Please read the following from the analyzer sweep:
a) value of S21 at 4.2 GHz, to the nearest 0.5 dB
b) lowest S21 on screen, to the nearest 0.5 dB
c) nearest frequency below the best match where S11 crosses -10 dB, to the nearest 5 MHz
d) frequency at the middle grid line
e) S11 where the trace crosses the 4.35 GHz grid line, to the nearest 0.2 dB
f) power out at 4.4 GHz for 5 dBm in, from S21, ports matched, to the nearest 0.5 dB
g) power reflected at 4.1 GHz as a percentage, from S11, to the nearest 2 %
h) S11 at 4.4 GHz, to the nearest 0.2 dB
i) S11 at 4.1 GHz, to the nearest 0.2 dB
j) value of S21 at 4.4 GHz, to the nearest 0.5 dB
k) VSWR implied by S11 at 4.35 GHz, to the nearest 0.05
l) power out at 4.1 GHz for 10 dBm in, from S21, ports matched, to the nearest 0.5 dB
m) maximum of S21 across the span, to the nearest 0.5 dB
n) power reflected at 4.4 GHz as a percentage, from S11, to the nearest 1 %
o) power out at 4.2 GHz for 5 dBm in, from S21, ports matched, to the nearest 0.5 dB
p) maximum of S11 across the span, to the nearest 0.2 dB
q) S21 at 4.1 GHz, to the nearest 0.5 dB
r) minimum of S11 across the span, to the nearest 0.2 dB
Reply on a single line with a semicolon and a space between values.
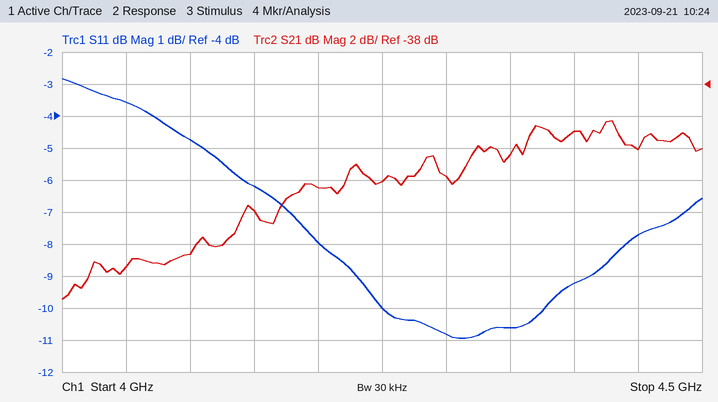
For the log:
-44.5 dB; -51.5 dB; 4.250 GHz; 4.25 GHz; -10.6 dB; -36.0 dBm; 34 %; -9.2 dB; -4.8 dB; -41.0 dB; 1.85; -38.5 dBm; -40.5 dB; 12 %; -39.5 dBm; -2.8 dB; -48.5 dB; -11.0 dB
